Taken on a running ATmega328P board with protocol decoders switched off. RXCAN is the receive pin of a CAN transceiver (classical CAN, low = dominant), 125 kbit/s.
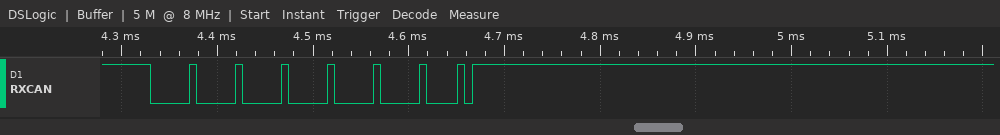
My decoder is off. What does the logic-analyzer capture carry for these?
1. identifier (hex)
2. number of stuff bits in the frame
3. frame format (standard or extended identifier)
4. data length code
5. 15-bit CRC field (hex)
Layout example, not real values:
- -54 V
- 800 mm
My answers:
- 0x000
- 6
- standard
- 0
- 0x0000
